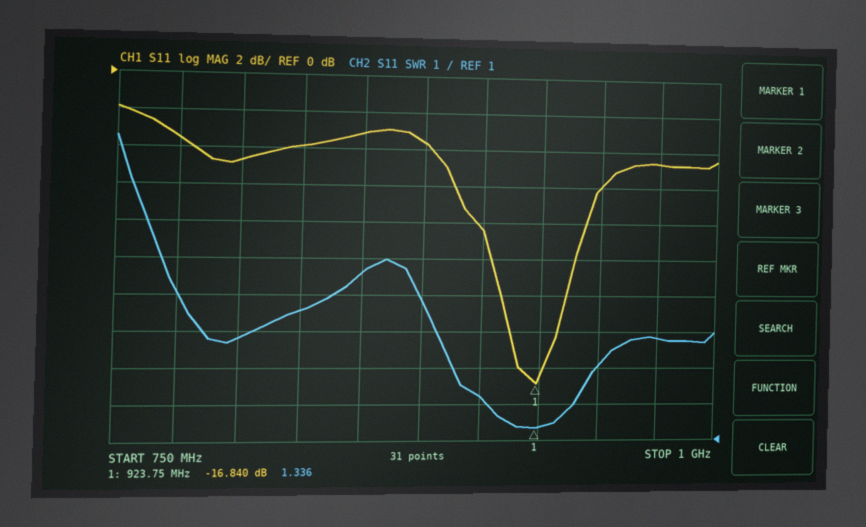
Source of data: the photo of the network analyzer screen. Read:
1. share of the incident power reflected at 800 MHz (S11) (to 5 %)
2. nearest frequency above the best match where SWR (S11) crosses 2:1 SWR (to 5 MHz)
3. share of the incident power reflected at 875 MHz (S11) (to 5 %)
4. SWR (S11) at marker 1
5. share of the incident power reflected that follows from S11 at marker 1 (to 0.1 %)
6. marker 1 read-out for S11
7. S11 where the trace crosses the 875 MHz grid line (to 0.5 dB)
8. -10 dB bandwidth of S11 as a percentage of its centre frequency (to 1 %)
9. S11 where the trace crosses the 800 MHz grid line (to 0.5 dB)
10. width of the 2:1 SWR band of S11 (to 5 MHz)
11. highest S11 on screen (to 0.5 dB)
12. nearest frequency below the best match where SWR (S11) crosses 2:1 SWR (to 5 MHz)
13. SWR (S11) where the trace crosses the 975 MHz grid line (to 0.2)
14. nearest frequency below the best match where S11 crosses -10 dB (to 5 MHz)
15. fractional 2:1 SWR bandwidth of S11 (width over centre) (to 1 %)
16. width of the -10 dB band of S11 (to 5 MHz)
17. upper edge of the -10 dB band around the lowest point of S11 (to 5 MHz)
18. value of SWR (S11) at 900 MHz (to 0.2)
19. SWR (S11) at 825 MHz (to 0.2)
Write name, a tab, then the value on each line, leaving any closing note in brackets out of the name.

share of the incident power reflected at 800 MHz (S11)	35 %
nearest frequency above the best match where SWR (S11) crosses 2:1 SWR	940 MHz
share of the incident power reflected at 875 MHz (S11)	45 %
SWR (S11) at marker 1	1.336
share of the incident power reflected that follows from S11 at marker 1	2.1 %
marker 1 read-out for S11	-16.840 dB
S11 where the trace crosses the 875 MHz grid line	-3.5 dB
-10 dB bandwidth of S11 as a percentage of its centre frequency	4 %
S11 where the trace crosses the 800 MHz grid line	-4.5 dB
width of the 2:1 SWR band of S11	35 MHz
highest S11 on screen	-2.0 dB
nearest frequency below the best match where SWR (S11) crosses 2:1 SWR	905 MHz
SWR (S11) where the trace crosses the 975 MHz grid line	3.8
nearest frequency below the best match where S11 crosses -10 dB	905 MHz
fractional 2:1 SWR bandwidth of S11 (width over centre)	4 %
width of the -10 dB band of S11	35 MHz
upper edge of the -10 dB band around the lowest point of S11	940 MHz
value of SWR (S11) at 900 MHz	2.2
SWR (S11) at 825 MHz	4.6
